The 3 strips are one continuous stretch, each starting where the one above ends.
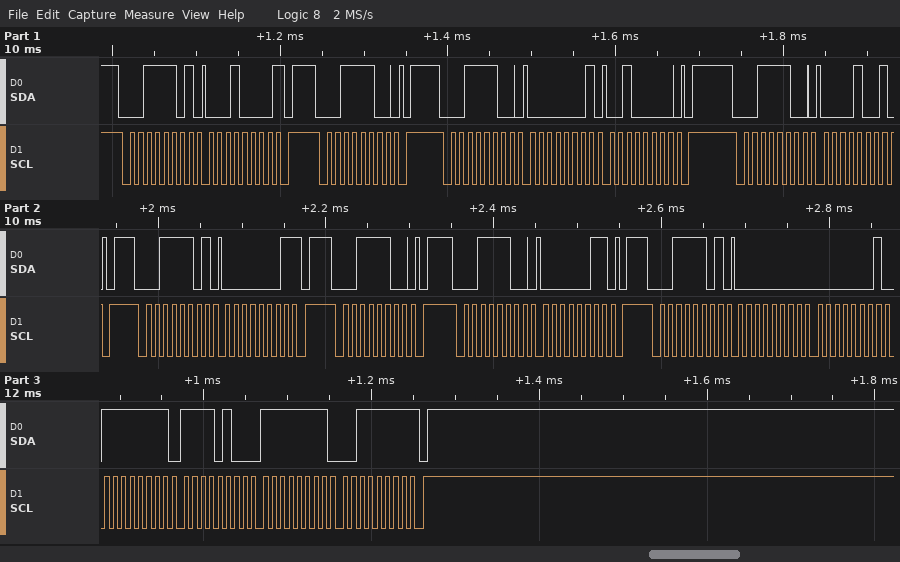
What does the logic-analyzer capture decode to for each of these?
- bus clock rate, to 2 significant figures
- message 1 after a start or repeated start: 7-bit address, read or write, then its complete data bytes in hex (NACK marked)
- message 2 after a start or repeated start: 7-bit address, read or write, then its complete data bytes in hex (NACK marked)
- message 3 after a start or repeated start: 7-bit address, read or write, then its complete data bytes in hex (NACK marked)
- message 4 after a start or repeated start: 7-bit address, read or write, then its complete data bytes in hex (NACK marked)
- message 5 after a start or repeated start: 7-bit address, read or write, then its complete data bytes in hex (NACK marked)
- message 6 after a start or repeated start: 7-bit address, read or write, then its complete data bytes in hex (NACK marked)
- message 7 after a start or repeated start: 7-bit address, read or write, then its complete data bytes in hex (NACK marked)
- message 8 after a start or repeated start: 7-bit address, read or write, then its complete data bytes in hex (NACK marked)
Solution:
100 kHz
0x1E read: 10 NACK
0x1E write
0x1E write: 01 20
0x1E write: 09
0x1E read: 01 NACK
0x1E write
0x1E write: 03
0x1E read: 00 01 FF F4 FF 3F NACK
